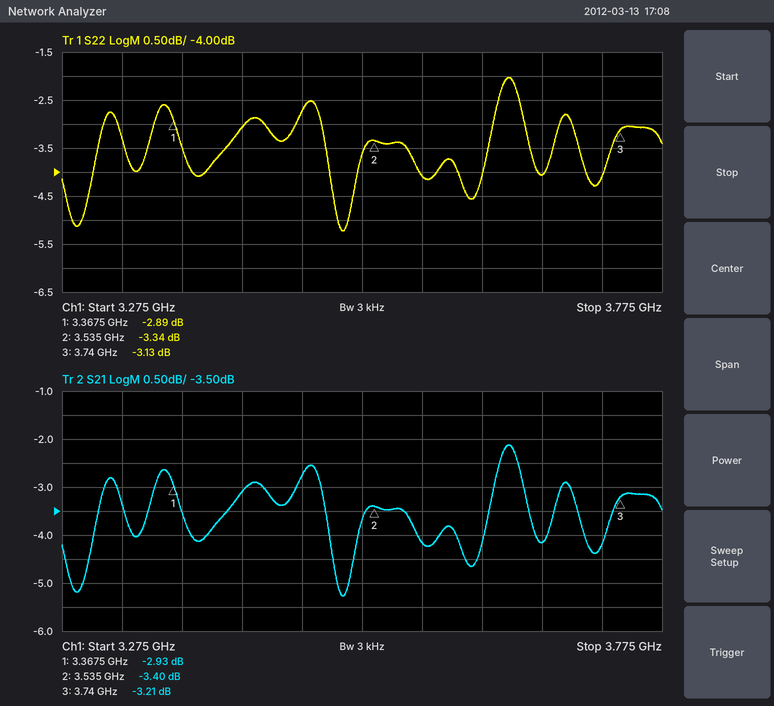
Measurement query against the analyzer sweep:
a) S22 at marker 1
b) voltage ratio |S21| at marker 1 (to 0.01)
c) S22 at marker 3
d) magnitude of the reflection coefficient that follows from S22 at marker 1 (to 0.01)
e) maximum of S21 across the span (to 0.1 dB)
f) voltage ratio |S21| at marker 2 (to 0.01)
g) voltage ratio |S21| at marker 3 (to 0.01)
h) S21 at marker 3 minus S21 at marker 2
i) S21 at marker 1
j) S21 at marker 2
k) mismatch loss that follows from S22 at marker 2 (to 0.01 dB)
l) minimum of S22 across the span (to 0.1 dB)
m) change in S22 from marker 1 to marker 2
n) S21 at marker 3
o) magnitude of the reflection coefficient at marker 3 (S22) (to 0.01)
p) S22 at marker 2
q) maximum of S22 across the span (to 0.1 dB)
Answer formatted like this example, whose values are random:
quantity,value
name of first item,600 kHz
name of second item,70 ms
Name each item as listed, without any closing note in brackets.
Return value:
quantity,value
S22 at marker 1,-2.89 dB
voltage ratio |S21| at marker 1,0.71
S22 at marker 3,-3.13 dB
magnitude of the reflection coefficient that follows from S22 at marker 1,0.72
maximum of S21 across the span,-2.1 dB
voltage ratio |S21| at marker 2,0.68
voltage ratio |S21| at marker 3,0.69
S21 at marker 3 minus S21 at marker 2,0.19 dB
S21 at marker 1,-2.93 dB
S21 at marker 2,-3.40 dB
mismatch loss that follows from S22 at marker 2,2.70 dB
minimum of S22 across the span,-5.2 dB
change in S22 from marker 1 to marker 2,-0.45 dB
S21 at marker 3,-3.21 dB
magnitude of the reflection coefficient at marker 3 (S22),0.70
S22 at marker 2,-3.34 dB
maximum of S22 across the span,-2.0 dB
